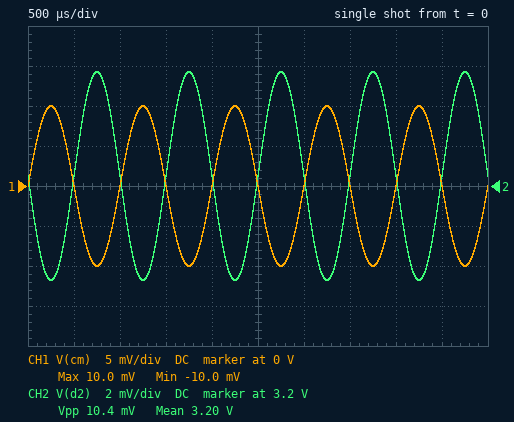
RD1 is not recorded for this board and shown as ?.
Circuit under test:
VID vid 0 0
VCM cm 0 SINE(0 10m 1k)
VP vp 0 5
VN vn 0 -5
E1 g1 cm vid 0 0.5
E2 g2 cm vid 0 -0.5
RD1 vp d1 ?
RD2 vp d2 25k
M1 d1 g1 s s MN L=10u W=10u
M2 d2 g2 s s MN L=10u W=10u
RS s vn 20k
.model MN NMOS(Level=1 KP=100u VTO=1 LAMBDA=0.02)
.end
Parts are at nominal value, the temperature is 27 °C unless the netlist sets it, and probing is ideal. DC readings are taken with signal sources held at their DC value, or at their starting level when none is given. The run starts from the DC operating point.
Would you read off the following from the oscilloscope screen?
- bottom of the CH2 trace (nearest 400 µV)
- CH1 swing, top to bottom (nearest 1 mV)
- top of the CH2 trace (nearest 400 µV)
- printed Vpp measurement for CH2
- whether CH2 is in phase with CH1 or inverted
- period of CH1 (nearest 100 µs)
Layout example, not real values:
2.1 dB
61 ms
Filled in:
3.1952 V
20 mV
3.2056 V
10.4 mV
inverted
1.0 ms
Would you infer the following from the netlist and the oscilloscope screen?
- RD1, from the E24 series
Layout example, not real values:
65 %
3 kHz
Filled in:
36 kΩ
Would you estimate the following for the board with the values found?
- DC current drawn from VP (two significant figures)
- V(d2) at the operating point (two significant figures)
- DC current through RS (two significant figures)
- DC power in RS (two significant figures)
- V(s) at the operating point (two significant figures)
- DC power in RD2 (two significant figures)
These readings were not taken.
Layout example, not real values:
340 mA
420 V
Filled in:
140 µA
3.2 V
140 µA
410 µW
-2.1 V
130 µW
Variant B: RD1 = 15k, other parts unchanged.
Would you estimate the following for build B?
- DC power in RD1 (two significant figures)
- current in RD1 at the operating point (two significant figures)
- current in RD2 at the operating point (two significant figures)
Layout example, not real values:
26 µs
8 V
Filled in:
78 µW
72 µA
71 µA
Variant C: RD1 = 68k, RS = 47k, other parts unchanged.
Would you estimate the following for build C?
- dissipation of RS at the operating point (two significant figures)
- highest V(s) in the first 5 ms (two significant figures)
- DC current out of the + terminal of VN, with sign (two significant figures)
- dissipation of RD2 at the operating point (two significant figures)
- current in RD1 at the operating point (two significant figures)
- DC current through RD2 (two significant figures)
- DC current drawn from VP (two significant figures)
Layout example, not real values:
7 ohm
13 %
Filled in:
220 µW
-1.8 V
-68 µA
30 µW
34 µA
35 µA
68 µA
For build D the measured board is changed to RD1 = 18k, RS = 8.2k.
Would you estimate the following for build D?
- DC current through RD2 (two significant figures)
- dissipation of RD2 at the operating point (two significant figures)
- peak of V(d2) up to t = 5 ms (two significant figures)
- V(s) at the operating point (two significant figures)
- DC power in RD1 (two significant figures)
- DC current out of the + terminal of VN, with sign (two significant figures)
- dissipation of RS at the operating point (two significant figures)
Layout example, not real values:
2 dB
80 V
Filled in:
140 µA
510 µW
1.4 V
-2.6 V
380 µW
-290 µA
690 µW
